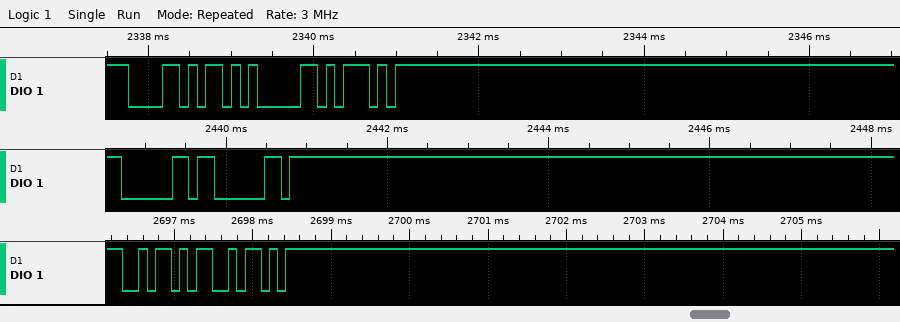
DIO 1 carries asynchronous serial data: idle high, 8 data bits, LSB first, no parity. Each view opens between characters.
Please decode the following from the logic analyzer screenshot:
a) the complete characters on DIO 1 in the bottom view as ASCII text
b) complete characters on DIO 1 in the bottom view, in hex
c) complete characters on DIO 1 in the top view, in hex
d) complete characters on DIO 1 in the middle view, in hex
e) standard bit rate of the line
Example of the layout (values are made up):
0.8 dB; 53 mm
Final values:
"ZZ"; 5A, 5A; 58, 05, 5D; 60, 60; 9600 baud
